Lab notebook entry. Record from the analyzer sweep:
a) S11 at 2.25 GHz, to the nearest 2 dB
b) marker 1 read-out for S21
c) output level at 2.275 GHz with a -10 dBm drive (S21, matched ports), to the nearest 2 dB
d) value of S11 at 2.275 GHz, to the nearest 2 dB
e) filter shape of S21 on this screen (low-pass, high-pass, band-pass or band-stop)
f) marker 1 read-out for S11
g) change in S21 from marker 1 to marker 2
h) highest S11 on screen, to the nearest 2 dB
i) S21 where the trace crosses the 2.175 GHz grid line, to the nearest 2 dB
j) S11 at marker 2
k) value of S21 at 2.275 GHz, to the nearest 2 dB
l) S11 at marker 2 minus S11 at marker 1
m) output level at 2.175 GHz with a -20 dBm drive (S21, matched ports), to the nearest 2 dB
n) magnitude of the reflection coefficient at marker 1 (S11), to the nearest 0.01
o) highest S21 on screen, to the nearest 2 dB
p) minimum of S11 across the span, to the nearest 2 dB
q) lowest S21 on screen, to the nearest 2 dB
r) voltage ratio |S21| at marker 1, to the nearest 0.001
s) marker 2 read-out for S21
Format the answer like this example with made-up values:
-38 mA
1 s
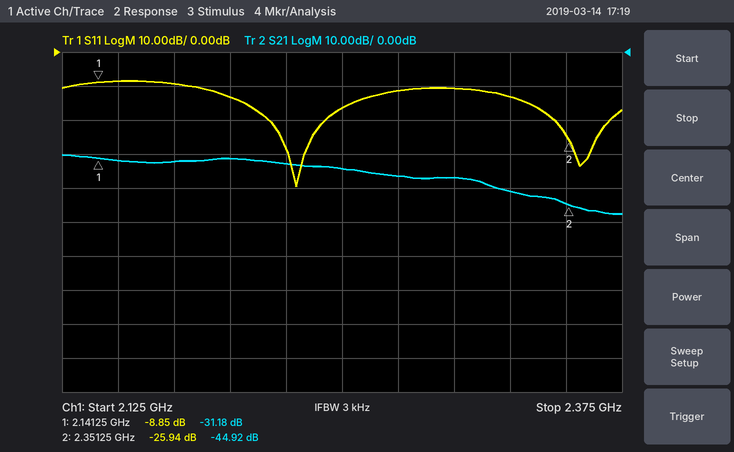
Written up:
-16 dB
-31.18 dB
-46 dBm
-12 dB
low-pass
-8.85 dB
-13.74 dB
-8 dB
-32 dB
-25.94 dB
-36 dB
-17.09 dB
-52 dBm
0.36
-30 dB
-40 dB
-48 dB
0.028
-44.92 dB
